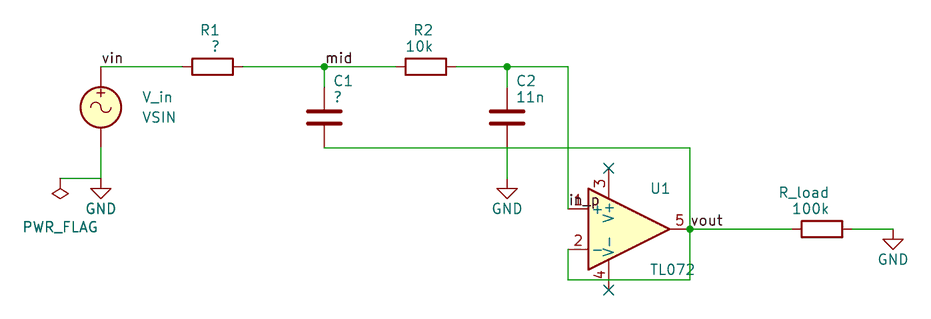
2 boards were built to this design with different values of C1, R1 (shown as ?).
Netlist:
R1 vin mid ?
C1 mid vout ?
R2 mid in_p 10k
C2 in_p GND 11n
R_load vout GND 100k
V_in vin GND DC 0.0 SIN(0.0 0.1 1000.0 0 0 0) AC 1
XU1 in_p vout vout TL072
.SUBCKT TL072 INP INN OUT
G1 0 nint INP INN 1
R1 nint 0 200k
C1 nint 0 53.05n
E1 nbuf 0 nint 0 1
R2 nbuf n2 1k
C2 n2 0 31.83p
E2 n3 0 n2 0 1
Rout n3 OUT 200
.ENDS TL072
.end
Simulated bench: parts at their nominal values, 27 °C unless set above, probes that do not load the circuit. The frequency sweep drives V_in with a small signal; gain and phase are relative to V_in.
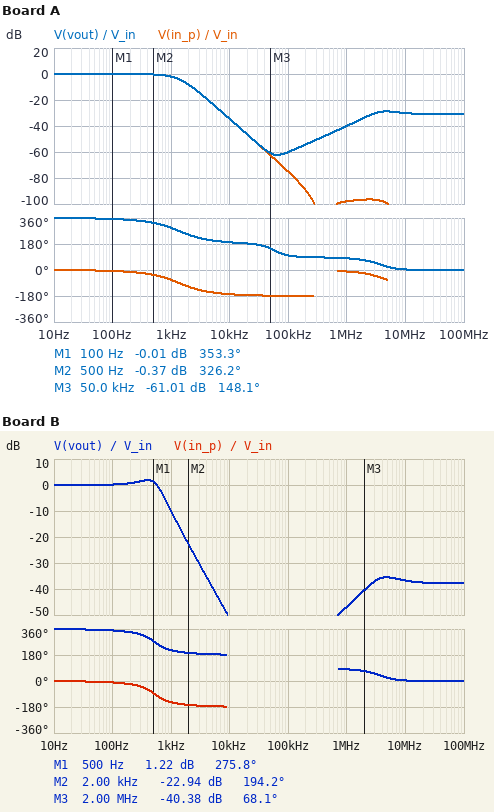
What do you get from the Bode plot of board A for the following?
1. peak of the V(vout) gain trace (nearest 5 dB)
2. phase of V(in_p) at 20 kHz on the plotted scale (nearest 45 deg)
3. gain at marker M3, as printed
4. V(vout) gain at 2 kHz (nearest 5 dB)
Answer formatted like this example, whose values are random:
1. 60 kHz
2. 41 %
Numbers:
1. 0 dB
2. -180 deg
3. -61.01 dB
4. -10 dB
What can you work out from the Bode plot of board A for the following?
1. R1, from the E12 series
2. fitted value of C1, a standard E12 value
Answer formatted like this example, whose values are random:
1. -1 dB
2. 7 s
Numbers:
1. 6.8 kΩ
2. 18 nF
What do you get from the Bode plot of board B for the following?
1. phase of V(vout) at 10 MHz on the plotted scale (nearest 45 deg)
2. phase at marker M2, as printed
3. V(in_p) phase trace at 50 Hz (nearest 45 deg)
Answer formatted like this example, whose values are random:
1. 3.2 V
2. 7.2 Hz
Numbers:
1. 0 deg
2. 194.2 deg
3. 0 deg
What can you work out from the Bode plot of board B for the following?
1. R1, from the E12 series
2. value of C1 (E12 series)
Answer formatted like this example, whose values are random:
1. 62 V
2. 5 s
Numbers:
1. 15 kΩ
2. 56 nF
